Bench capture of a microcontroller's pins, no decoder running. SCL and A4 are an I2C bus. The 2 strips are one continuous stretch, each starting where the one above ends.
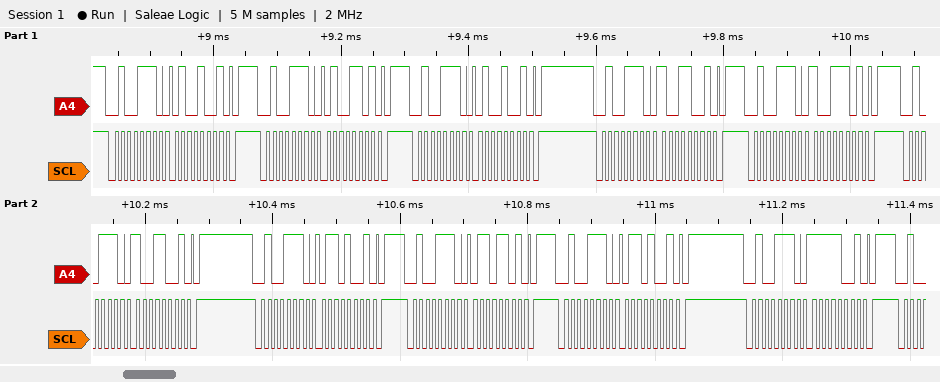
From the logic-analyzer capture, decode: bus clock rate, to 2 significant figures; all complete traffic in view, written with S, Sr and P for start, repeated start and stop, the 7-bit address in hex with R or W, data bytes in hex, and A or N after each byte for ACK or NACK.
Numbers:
100 kHz
S 27W A 49 A P S 27W A 4D A P S 27W A 49 A P S 27W A 99 A P S 27W A 9D A P S 27W A 99 A P S 27W A 69 A P S 27W A 6D A P S 27W A 69 A P S 27W A F9 A P
